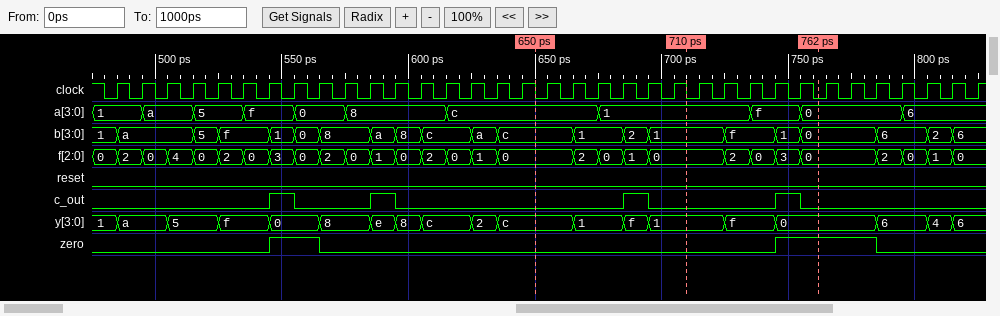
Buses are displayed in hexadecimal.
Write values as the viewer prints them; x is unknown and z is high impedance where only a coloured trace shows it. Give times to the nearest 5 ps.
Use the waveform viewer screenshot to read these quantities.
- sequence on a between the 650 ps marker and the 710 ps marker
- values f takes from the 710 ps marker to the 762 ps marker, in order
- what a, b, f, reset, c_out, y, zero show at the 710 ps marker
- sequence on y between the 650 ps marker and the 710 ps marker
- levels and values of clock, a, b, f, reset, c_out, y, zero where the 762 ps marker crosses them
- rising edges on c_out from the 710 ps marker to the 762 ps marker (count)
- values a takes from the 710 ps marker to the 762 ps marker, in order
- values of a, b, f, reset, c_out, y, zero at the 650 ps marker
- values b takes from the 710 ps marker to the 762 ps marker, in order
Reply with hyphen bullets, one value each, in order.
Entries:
- c, 1
- 0, 2, 0, 3, 0
- a=1, b=1, f=0, reset=0, c_out=0, y=1, zero=0
- c, 1, f, 1
- clock=0, a=0, b=0, f=0, reset=0, c_out=0, y=0, zero=1
- 1
- 1, f, 0
- a=c, b=c, f=0, reset=0, c_out=0, y=c, zero=0
- 1, f, 1, 0
